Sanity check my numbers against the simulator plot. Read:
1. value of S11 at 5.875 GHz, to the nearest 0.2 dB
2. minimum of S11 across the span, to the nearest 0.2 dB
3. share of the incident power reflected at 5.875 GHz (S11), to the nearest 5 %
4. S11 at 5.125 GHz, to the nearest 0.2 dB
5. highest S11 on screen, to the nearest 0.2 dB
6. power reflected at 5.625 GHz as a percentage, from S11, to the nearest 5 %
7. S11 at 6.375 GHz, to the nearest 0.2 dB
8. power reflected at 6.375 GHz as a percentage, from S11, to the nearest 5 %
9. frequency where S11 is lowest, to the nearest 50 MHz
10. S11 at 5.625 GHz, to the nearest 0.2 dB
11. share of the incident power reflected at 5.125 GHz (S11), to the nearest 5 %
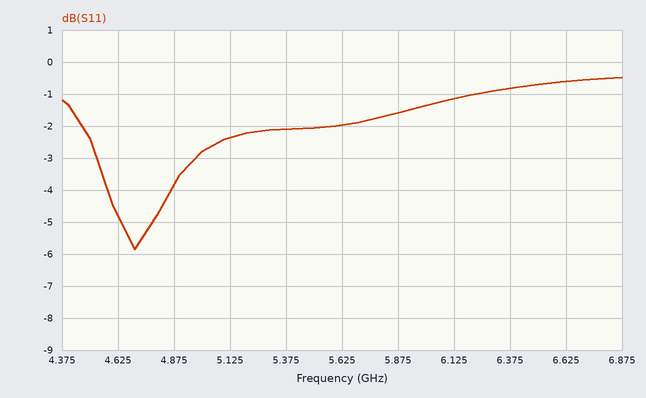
-1.6 dB
-5.8 dB
70 %
-2.4 dB
-0.4 dB
65 %
-0.8 dB
85 %
4.70 GHz
-2.0 dB
60 %
